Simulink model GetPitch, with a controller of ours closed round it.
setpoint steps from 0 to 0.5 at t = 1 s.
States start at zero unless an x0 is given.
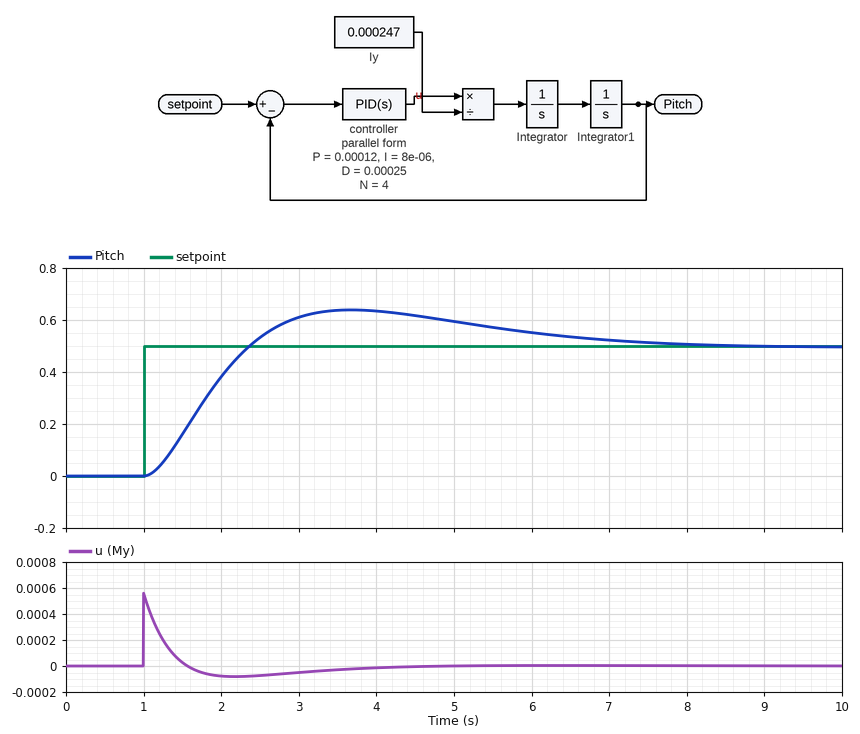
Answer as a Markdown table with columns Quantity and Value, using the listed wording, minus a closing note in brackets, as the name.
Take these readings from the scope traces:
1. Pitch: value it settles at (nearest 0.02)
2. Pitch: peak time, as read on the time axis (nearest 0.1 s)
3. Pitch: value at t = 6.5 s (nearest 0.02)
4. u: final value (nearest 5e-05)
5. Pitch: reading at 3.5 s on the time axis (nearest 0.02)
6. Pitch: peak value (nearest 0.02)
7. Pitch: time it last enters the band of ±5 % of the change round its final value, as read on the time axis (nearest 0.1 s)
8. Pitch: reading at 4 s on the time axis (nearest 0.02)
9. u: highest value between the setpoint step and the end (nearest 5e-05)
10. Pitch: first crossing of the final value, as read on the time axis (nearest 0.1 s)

| Quantity | Value |
|---|---|
| Pitch: value it settles at | 0.50 |
| Pitch: peak time, as read on the time axis | 3.7 s |
| Pitch: value at t = 6.5 s | 0.54 |
| u: final value | 0.00000 |
| Pitch: reading at 3.5 s on the time axis | 0.64 |
| Pitch: peak value | 0.64 |
| Pitch: time it last enters the band of ±5 % of the change round its final value, as read on the time axis | 6.9 s |
| Pitch: reading at 4 s on the time axis | 0.64 |
| u: highest value between the setpoint step and the end | 0.00055 |
| Pitch: first crossing of the final value, as read on the time axis | 2.4 s |
